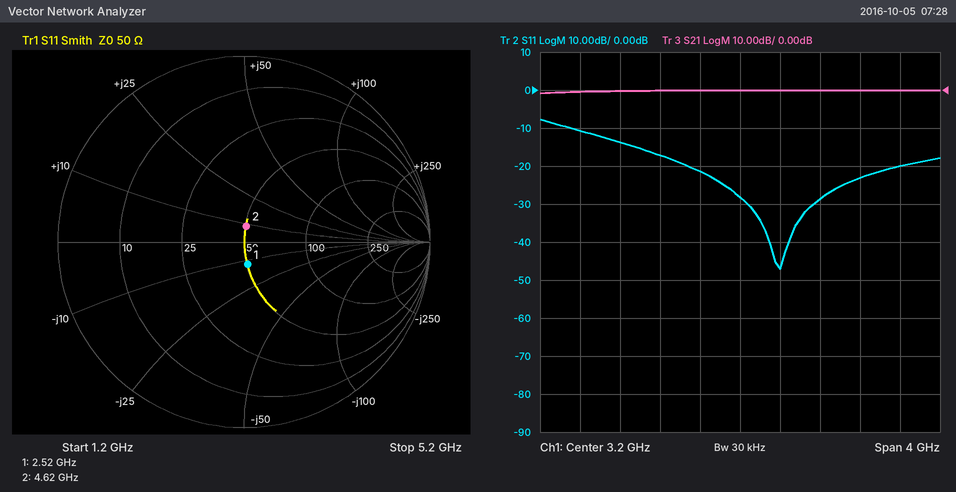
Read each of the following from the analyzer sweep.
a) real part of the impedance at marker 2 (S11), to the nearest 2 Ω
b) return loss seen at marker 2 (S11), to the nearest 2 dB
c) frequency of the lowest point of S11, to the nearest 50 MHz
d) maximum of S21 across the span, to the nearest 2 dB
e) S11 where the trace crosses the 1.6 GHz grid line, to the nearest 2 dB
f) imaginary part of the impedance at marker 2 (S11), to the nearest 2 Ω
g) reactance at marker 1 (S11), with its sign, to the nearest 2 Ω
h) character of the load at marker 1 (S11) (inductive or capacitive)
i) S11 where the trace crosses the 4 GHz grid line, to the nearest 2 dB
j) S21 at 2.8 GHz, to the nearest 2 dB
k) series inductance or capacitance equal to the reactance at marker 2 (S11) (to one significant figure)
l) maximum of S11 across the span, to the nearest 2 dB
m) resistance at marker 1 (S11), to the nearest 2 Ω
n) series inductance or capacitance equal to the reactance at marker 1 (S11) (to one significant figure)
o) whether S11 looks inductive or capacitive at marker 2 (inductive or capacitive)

50 Ω
22 dB
3.60 GHz
0 dB
-10 dB
+8 Ω
-12 Ω
capacitive
-28 dB
0 dB
300 pH
-8 dB
50 Ω
5 pF
inductive
